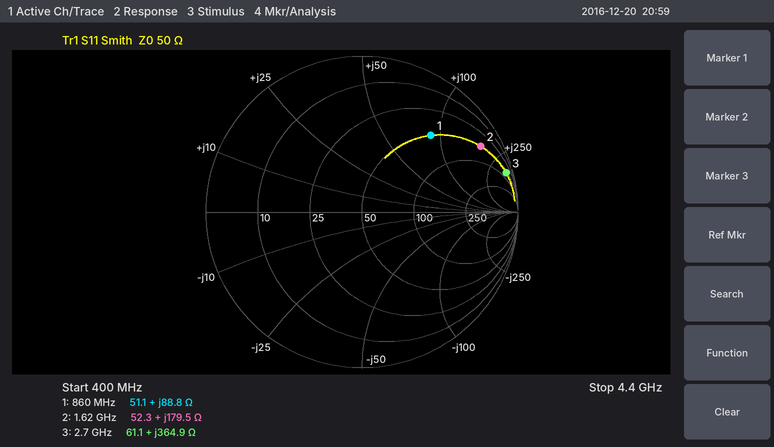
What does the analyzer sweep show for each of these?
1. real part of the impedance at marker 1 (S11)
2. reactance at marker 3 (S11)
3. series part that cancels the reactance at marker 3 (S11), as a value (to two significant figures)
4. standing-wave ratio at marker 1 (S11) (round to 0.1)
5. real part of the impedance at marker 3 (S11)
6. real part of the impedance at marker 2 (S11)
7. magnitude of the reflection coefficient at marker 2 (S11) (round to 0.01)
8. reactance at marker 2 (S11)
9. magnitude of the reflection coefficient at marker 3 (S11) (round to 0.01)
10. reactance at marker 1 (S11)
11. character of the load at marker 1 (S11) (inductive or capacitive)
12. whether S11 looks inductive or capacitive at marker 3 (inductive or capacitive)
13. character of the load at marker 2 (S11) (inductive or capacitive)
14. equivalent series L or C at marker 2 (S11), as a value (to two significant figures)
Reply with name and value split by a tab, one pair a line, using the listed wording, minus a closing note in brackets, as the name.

real part of the impedance at marker 1	51.1 Ω
reactance at marker 3	+364.9 Ω
series part that cancels the reactance at marker 3 (S11), as a value	160 fF
standing-wave ratio at marker 1 (S11)	4.9
real part of the impedance at marker 3	61.1 Ω
real part of the impedance at marker 2	52.3 Ω
magnitude of the reflection coefficient at marker 2 (S11)	0.87
reactance at marker 2	+179.5 Ω
magnitude of the reflection coefficient at marker 3 (S11)	0.96
reactance at marker 1	+88.8 Ω
character of the load at marker 1 (S11)	inductive
whether S11 looks inductive or capacitive at marker 3	inductive
character of the load at marker 2 (S11)	inductive
equivalent series L or C at marker 2 (S11), as a value	18 nH
